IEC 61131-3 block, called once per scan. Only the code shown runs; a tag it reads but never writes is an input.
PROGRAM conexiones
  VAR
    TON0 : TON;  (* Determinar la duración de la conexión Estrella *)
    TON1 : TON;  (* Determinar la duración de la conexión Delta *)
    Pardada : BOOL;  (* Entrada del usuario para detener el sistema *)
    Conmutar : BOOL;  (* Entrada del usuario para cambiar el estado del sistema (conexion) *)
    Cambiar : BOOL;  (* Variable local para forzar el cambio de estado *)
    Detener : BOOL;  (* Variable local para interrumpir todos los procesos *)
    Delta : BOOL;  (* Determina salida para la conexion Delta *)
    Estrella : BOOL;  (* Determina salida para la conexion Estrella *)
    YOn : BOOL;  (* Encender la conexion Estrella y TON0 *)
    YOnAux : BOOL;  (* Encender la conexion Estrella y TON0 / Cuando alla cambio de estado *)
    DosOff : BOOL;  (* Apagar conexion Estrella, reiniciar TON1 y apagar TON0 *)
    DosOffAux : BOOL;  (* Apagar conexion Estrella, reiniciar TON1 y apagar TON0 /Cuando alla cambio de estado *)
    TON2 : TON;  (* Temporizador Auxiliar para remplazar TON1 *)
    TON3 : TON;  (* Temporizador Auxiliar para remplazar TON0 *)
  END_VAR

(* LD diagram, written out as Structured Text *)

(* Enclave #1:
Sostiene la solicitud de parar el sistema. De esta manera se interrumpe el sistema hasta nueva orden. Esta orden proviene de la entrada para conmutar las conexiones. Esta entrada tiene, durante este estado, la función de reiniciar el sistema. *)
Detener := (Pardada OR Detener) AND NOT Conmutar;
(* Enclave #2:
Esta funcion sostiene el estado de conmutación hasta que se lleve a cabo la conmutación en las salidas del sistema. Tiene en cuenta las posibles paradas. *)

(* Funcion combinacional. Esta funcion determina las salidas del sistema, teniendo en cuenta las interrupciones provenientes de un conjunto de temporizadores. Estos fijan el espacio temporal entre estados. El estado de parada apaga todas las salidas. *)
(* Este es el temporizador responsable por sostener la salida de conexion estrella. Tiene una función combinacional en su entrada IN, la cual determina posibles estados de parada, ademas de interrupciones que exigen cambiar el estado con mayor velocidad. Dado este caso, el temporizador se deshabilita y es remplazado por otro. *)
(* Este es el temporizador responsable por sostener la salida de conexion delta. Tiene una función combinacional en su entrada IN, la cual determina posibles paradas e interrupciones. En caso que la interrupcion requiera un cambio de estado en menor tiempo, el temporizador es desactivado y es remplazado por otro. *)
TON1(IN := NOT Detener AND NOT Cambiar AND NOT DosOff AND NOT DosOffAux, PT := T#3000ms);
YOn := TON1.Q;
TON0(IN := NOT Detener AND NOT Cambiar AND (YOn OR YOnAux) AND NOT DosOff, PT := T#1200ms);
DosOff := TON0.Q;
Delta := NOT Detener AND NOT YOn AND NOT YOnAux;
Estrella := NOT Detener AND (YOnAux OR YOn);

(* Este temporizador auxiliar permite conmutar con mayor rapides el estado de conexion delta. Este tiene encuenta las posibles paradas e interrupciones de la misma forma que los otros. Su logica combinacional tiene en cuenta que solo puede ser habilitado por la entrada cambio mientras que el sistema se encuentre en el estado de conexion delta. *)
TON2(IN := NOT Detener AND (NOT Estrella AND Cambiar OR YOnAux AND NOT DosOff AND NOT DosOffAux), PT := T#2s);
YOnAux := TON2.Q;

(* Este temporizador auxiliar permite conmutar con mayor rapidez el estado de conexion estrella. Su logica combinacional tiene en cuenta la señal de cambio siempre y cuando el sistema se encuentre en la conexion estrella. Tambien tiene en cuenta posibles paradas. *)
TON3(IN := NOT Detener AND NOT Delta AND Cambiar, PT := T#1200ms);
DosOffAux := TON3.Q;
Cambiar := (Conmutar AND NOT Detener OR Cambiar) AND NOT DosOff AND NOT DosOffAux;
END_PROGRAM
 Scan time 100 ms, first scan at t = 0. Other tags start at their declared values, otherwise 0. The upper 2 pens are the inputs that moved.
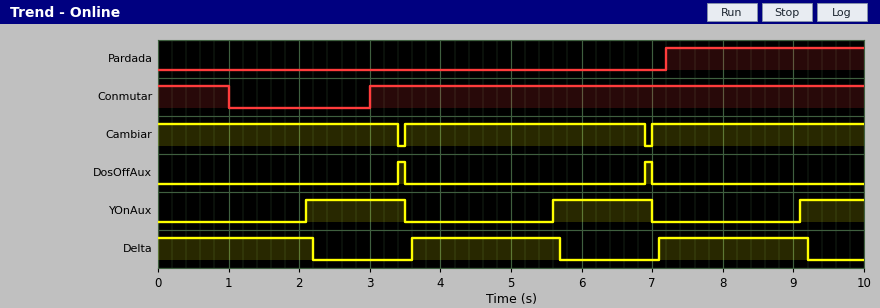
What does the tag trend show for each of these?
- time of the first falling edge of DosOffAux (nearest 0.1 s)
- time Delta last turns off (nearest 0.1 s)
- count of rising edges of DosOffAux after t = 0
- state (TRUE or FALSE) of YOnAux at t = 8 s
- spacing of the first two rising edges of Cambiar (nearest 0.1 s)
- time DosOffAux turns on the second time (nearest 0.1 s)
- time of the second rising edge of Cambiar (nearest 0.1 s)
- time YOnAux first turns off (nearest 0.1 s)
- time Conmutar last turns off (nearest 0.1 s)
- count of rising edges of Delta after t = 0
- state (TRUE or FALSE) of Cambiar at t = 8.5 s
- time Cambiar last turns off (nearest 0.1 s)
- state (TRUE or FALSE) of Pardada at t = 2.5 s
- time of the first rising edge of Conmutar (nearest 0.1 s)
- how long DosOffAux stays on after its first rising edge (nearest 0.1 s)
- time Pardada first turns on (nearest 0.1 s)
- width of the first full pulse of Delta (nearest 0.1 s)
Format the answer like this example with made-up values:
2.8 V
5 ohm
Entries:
3.5 s
9.2 s
2
FALSE
3.5 s
6.9 s
7.0 s
3.5 s
1.0 s
2
TRUE
6.9 s
FALSE
3.0 s
0.1 s
7.2 s
2.1 s
